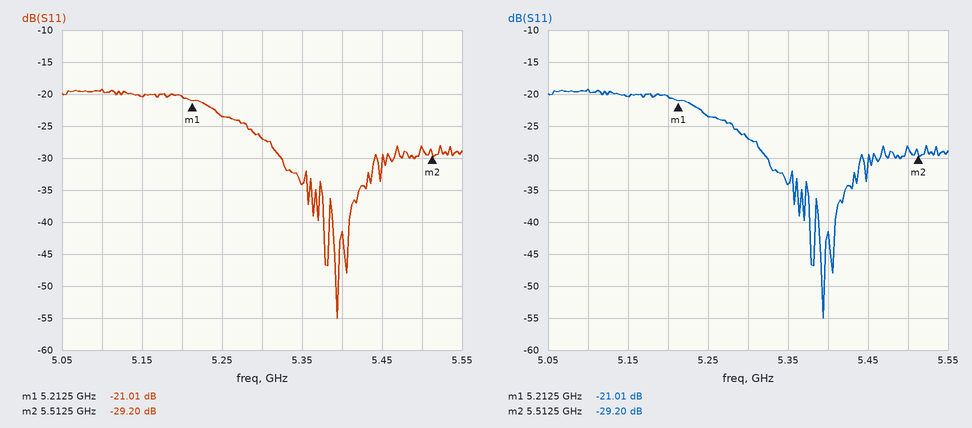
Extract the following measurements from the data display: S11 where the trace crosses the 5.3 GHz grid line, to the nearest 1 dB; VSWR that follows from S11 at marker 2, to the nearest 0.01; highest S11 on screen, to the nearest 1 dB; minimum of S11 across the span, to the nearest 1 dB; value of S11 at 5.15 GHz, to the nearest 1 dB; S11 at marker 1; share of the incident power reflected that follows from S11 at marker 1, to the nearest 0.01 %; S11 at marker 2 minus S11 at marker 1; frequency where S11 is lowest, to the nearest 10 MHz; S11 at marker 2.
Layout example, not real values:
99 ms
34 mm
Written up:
-27 dB
1.07
-19 dB
-55 dB
-20 dB
-21.01 dB
0.79 %
-8.19 dB
5.39 GHz
-29.20 dB
